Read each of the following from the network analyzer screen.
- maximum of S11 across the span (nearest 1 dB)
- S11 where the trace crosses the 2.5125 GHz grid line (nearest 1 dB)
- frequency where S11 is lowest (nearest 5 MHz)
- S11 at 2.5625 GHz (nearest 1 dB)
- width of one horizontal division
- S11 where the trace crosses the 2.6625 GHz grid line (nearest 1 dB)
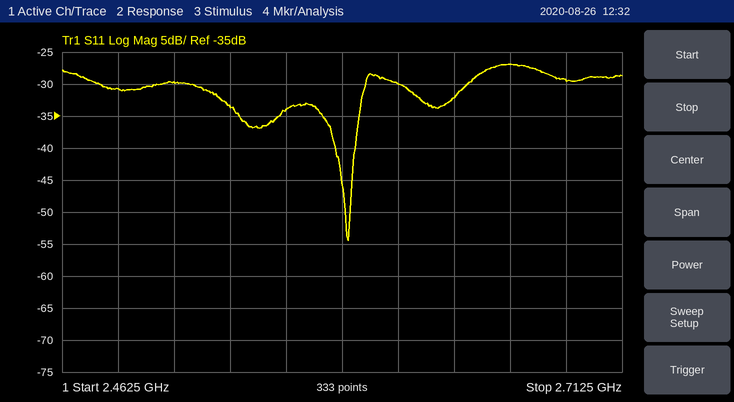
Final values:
-27 dB
-30 dB
2.590 GHz
-34 dB
25 MHz
-27 dB
